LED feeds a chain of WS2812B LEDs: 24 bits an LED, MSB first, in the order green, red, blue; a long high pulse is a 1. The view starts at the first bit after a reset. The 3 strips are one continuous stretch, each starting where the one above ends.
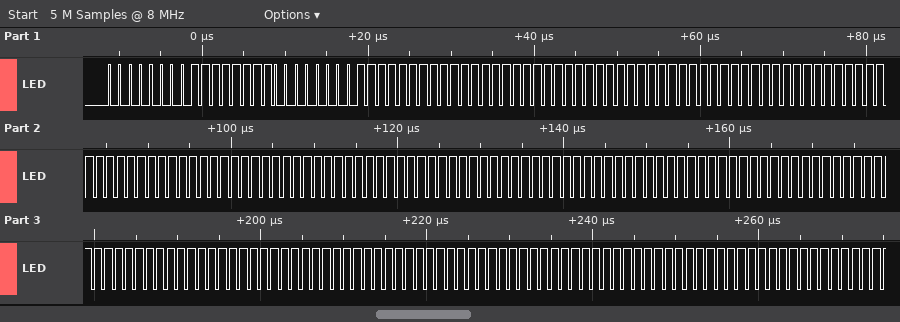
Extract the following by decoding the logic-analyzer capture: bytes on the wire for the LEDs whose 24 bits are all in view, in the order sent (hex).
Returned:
00 FF 00 FF FF FF FF FF FF FF FF FF FF FF FF FF FF FF FF FF FF FF FF FF FF FF FF
